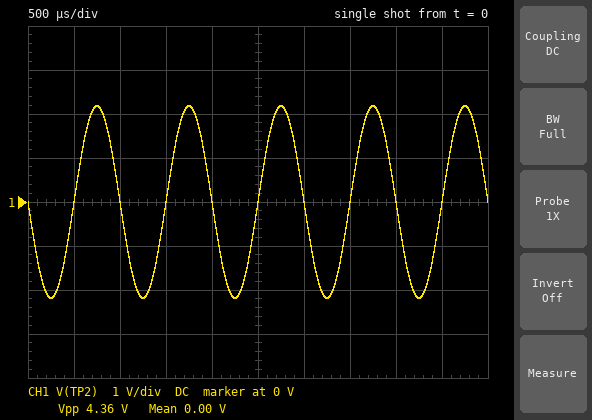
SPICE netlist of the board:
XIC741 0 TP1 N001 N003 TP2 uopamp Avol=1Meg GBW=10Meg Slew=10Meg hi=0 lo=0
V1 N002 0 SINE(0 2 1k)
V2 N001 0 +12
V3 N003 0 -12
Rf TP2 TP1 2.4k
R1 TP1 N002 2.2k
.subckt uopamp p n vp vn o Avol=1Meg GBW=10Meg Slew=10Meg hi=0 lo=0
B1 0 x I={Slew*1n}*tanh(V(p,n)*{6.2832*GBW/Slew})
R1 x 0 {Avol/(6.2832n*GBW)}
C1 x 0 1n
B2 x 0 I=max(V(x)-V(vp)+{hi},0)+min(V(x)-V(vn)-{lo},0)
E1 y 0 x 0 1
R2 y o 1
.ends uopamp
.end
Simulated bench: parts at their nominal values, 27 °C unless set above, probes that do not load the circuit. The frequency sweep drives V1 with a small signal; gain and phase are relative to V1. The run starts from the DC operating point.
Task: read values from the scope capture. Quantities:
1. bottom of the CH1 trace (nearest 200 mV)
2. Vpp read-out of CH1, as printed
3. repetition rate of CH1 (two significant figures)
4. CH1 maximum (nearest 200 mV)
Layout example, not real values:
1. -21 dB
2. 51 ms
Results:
1. -2.2 V
2. 4.36 V
3. 1.0 kHz
4. 2.2 V
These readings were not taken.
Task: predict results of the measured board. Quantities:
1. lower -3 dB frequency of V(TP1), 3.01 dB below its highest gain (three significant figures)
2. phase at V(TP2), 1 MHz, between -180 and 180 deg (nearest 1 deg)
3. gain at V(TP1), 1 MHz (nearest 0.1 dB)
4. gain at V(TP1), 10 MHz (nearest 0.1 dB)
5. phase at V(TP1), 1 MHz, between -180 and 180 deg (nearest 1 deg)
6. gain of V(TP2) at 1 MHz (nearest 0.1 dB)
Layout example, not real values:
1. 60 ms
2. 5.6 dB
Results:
1. 4.78 MHz
2. 168 deg
3. -19.4 dB
4. -6.5 dB
5. 78 deg
6. 0.6 dB
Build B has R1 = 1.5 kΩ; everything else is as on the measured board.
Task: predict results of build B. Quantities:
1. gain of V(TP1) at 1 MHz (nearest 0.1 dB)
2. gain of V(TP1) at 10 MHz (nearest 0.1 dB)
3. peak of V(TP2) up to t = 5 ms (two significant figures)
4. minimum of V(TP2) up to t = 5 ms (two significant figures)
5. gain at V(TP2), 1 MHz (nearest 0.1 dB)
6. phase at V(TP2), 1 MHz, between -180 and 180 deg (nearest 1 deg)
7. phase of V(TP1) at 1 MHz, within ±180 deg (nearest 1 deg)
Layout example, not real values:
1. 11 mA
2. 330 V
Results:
1. -16.2 dB
2. -4.8 dB
3. 3.2 V
4. -3.2 V
5. 3.8 dB
6. 165 deg
7. 75 deg
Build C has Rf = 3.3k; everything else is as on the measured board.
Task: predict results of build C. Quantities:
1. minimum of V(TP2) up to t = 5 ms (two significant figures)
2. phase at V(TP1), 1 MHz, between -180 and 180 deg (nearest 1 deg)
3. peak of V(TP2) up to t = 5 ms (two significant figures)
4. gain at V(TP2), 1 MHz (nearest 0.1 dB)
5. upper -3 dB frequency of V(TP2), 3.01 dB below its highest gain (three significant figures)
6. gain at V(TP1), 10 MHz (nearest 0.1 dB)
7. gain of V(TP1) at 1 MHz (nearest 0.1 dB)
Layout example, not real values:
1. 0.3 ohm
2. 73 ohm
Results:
1. -3.0 V
2. 76 deg
3. 3.0 V
4. 3.3 dB
5. 4.00 MHz
6. -5.1 dB
7. -16.7 dB
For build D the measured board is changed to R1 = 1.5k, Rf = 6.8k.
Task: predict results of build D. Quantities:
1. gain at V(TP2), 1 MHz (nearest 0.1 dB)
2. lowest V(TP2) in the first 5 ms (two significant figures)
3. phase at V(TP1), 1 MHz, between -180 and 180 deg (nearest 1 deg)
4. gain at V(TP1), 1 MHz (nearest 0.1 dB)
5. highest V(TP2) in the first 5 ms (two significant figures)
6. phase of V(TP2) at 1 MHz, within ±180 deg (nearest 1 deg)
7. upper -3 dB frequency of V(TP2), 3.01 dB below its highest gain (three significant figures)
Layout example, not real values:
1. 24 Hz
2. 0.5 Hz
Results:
1. 12.0 dB
2. -9.1 V
3. 61 deg
4. -8.0 dB
5. 9.1 V
6. 151 deg
7. 1.81 MHz
